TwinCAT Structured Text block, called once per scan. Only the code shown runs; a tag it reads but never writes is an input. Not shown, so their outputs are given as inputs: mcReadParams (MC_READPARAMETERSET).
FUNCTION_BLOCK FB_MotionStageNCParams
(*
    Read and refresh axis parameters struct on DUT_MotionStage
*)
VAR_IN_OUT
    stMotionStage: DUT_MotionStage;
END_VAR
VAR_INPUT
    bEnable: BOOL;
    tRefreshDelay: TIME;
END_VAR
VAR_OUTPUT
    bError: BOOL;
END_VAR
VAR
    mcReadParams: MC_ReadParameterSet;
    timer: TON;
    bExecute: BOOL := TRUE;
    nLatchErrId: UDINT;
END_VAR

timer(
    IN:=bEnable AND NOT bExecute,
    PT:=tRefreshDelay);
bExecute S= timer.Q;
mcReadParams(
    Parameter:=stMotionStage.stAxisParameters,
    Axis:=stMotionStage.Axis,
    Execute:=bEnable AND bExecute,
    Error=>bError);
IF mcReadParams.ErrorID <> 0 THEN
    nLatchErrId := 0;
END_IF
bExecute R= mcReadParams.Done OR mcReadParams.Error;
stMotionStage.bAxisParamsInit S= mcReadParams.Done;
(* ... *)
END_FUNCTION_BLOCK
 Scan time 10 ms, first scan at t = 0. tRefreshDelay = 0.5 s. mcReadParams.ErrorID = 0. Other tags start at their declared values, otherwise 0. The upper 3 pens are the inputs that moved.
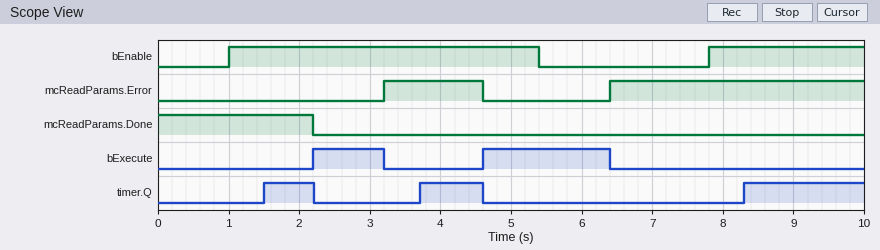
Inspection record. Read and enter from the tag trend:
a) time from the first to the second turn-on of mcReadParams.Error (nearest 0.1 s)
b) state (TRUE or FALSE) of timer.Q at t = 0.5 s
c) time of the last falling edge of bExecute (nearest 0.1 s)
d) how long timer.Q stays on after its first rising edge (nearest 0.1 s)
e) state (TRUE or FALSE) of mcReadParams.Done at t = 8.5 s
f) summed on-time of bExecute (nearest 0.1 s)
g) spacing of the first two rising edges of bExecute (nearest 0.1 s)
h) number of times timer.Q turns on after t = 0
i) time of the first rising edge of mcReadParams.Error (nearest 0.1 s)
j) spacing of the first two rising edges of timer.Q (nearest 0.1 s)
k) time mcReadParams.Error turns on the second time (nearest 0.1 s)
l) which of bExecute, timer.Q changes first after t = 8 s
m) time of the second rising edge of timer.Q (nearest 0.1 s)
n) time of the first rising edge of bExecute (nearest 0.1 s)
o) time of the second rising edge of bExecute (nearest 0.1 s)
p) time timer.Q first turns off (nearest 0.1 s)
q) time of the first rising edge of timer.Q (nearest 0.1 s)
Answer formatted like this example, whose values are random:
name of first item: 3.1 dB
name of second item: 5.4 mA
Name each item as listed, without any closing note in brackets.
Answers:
time from the first to the second turn-on of mcReadParams.Error: 3.2 s
state (TRUE or FALSE) of timer.Q at t = 0.5 s: FALSE
time of the last falling edge of bExecute: 6.4 s
how long timer.Q stays on after its first rising edge: 0.7 s
state (TRUE or FALSE) of mcReadParams.Done at t = 8.5 s: FALSE
summed on-time of bExecute: 2.8 s
spacing of the first two rising edges of bExecute: 2.4 s
number of times timer.Q turns on after t = 0: 3
time of the first rising edge of mcReadParams.Error: 3.2 s
spacing of the first two rising edges of timer.Q: 2.2 s
time mcReadParams.Error turns on the second time: 6.4 s
which of bExecute, timer.Q changes first after t = 8 s: timer.Q
time of the second rising edge of timer.Q: 3.7 s
time of the first rising edge of bExecute: 2.2 s
time of the second rising edge of bExecute: 4.6 s
time timer.Q first turns off: 2.2 s
time of the first rising edge of timer.Q: 1.5 s
